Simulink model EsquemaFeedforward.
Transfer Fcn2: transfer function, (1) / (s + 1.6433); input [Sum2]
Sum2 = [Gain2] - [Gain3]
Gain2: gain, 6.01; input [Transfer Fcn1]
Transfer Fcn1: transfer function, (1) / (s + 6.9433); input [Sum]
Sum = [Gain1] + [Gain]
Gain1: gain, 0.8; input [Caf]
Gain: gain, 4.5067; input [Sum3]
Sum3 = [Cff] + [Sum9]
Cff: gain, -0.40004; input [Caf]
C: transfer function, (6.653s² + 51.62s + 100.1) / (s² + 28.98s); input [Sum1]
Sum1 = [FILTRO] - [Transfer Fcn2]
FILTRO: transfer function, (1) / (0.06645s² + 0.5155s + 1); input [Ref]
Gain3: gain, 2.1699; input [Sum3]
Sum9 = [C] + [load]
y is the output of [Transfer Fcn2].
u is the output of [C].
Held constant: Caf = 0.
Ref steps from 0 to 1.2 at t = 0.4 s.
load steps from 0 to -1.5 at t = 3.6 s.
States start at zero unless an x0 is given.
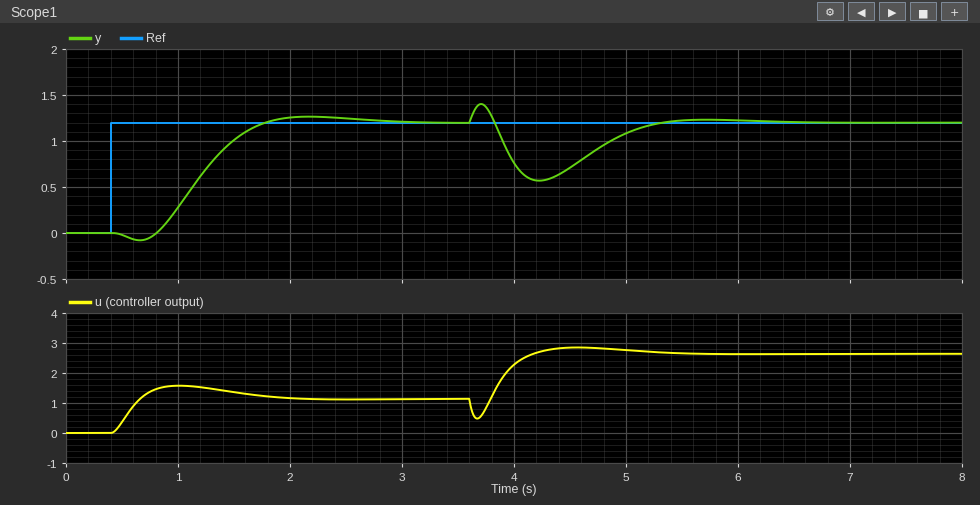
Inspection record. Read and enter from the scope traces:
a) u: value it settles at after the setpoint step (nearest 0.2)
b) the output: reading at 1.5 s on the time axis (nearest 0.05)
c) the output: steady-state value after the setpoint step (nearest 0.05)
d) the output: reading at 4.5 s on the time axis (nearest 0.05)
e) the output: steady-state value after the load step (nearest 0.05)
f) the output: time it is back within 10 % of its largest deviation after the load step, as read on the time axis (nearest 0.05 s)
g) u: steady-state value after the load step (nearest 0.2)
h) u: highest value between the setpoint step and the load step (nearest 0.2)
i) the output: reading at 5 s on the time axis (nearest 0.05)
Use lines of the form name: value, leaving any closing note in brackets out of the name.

u: value it settles at after the setpoint step: 1.2
the output: reading at 1.5 s on the time axis: 1.00
the output: steady-state value after the setpoint step: 1.20
the output: reading at 4.5 s on the time axis: 0.70
the output: steady-state value after the load step: 1.20
the output: time it is back within 10 % of its largest deviation after the load step, as read on the time axis: 5.10 s
u: steady-state value after the load step: 2.6
u: highest value between the setpoint step and the load step: 1.6
the output: reading at 5 s on the time axis: 1.10
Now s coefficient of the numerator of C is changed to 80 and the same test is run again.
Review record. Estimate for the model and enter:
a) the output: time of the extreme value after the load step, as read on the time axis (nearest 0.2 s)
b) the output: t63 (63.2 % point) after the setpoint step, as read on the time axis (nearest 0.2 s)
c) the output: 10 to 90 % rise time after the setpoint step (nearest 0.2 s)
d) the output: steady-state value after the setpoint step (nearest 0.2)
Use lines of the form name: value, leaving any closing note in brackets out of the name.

the output: time of the extreme value after the load step, as read on the time axis: 4.2 s
the output: t63 (63.2 % point) after the setpoint step, as read on the time axis: 1.2 s
the output: 10 to 90 % rise time after the setpoint step: 0.8 s
the output: steady-state value after the setpoint step: 1.2
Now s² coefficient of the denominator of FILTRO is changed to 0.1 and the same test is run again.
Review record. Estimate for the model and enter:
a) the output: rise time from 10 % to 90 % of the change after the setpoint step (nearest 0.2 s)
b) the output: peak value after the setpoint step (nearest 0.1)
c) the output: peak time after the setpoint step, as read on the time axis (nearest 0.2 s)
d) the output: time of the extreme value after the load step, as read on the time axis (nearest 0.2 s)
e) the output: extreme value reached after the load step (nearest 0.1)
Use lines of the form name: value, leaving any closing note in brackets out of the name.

the output: rise time from 10 % to 90 % of the change after the setpoint step: 0.6 s
the output: peak value after the setpoint step: 1.3
the output: peak time after the setpoint step, as read on the time axis: 2.2 s
the output: time of the extreme value after the load step, as read on the time axis: 4.2 s
the output: extreme value reached after the load step: 0.6
